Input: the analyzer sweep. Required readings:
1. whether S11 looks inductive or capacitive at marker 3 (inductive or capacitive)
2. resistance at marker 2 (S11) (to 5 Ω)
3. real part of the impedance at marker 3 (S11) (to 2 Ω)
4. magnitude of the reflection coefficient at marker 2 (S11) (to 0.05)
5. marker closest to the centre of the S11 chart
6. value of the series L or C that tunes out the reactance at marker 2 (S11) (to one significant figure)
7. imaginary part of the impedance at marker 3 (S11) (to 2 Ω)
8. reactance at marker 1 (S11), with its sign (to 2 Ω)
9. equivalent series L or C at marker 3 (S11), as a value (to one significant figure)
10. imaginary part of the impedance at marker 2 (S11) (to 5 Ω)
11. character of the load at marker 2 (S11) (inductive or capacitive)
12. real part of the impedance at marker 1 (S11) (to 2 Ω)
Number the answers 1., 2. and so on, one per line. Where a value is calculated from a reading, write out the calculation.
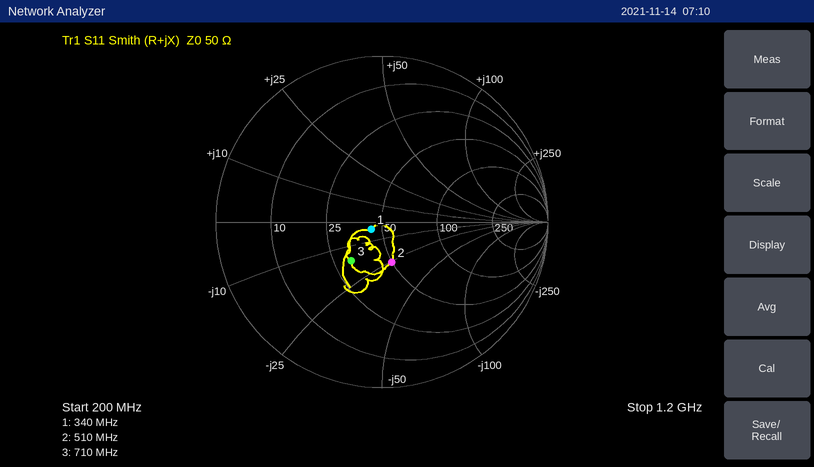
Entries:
1. capacitive
2. 50 Ω
3. 32 Ω
4. 0.25
5. marker 1
6. L = 25 Ω/(2π × 510 MHz) ≈ 8 nH
7. -16 Ω
8. -4 Ω
9. C = 1/(2π × 710 MHz × 16 Ω) ≈ 14.0 pF, so 10 pF to one significant figure
10. -25 Ω
11. capacitive
12. 44 Ω
